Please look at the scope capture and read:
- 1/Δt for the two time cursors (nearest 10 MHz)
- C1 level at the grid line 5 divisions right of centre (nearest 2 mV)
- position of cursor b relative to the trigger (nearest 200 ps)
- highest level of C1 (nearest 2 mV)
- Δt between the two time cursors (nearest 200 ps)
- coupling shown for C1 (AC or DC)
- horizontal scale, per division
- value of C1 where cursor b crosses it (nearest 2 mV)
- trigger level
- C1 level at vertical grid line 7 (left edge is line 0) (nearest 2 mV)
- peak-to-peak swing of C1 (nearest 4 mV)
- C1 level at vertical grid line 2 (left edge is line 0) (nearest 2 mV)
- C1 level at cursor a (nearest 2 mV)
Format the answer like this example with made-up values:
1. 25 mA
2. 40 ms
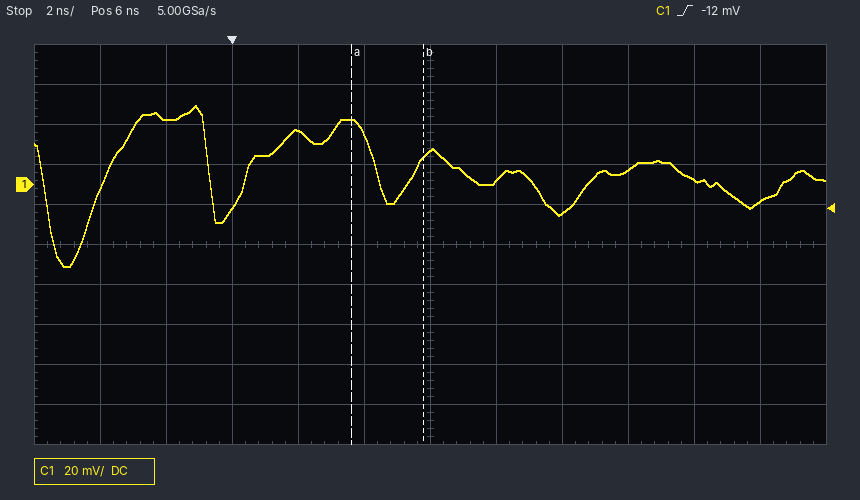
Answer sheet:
1. 450 MHz
2. -8 mV
3. +5.8 ns
4. 40 mV
5. 2.2 ns
6. DC
7. 2 ns
8. 14 mV
9. -12 mV
10. 2 mV
11. 80 mV
12. 32 mV
13. 32 mV
